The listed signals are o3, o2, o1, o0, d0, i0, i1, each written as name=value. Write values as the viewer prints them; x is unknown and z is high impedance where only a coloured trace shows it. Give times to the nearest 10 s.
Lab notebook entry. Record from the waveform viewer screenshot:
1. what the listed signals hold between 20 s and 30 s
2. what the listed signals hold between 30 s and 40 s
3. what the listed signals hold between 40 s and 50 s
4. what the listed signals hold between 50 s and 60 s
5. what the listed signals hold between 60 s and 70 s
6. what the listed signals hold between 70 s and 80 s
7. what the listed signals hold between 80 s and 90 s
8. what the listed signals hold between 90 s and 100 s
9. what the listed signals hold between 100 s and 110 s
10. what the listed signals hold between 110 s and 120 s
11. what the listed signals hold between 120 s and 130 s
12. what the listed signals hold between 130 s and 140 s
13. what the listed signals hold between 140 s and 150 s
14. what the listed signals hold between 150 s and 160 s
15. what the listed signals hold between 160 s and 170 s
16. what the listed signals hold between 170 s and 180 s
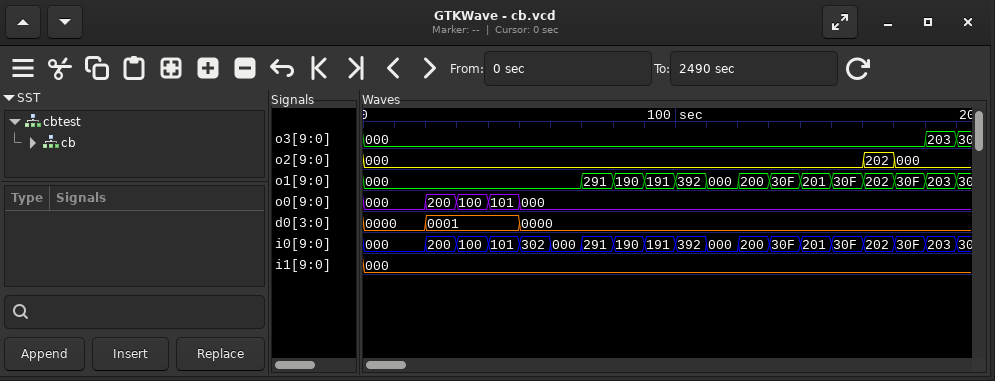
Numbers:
o3=000, o2=000, o1=000, o0=200, d0=0001, i0=200, i1=000
o3=000, o2=000, o1=000, o0=100, d0=0001, i0=100, i1=000
o3=000, o2=000, o1=000, o0=101, d0=0001, i0=101, i1=000
o3=000, o2=000, o1=000, o0=000, d0=0000, i0=302, i1=000
o3=000, o2=000, o1=000, o0=000, d0=0000, i0=000, i1=000
o3=000, o2=000, o1=291, o0=000, d0=0000, i0=291, i1=000
o3=000, o2=000, o1=190, o0=000, d0=0000, i0=190, i1=000
o3=000, o2=000, o1=191, o0=000, d0=0000, i0=191, i1=000
o3=000, o2=000, o1=392, o0=000, d0=0000, i0=392, i1=000
o3=000, o2=000, o1=000, o0=000, d0=0000, i0=000, i1=000
o3=000, o2=000, o1=200, o0=000, d0=0000, i0=200, i1=000
o3=000, o2=000, o1=30F, o0=000, d0=0000, i0=30F, i1=000
o3=000, o2=000, o1=201, o0=000, d0=0000, i0=201, i1=000
o3=000, o2=000, o1=30F, o0=000, d0=0000, i0=30F, i1=000
o3=000, o2=202, o1=202, o0=000, d0=0000, i0=202, i1=000
o3=000, o2=000, o1=30F, o0=000, d0=0000, i0=30F, i1=000
